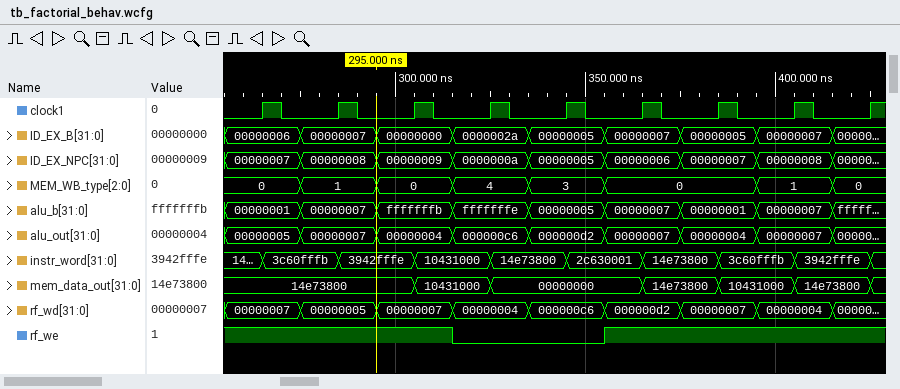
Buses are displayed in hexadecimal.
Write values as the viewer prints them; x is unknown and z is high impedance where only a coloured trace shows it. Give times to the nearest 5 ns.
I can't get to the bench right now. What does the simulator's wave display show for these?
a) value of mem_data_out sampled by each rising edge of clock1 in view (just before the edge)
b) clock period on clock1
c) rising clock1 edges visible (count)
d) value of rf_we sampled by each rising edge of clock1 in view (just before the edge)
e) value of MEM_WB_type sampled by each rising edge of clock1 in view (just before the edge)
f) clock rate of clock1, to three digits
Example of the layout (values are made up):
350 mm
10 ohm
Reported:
14e73800, 14e73800, 14e73800, 10431000, 00000000, 00000000, 14e73800, 10431000, 14e73800
20 ns
9
1 1 1 0 0 1 1 1 1
0, 1, 0, 4, 3, 0, 0, 1, 0
50.0 MHz
